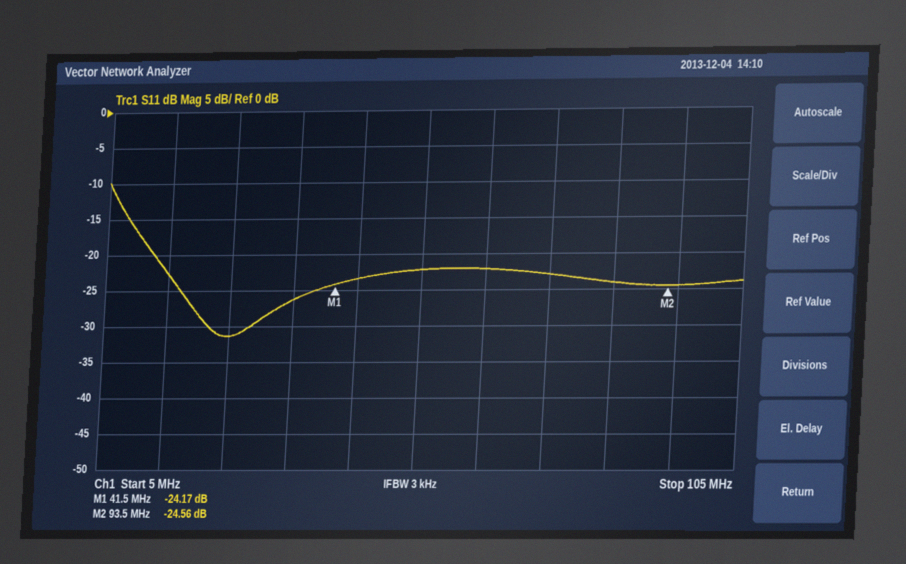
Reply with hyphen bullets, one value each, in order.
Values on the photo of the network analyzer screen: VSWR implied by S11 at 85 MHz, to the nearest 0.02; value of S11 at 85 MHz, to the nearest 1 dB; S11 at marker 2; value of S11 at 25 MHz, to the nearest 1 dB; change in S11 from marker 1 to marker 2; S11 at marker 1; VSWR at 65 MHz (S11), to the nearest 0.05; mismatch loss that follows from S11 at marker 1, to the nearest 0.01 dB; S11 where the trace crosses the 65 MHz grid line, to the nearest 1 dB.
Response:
- 1.14
- -24 dB
- -24.56 dB
- -31 dB
- -0.39 dB
- -24.17 dB
- 1.15
- 0.02 dB
- -22 dB
